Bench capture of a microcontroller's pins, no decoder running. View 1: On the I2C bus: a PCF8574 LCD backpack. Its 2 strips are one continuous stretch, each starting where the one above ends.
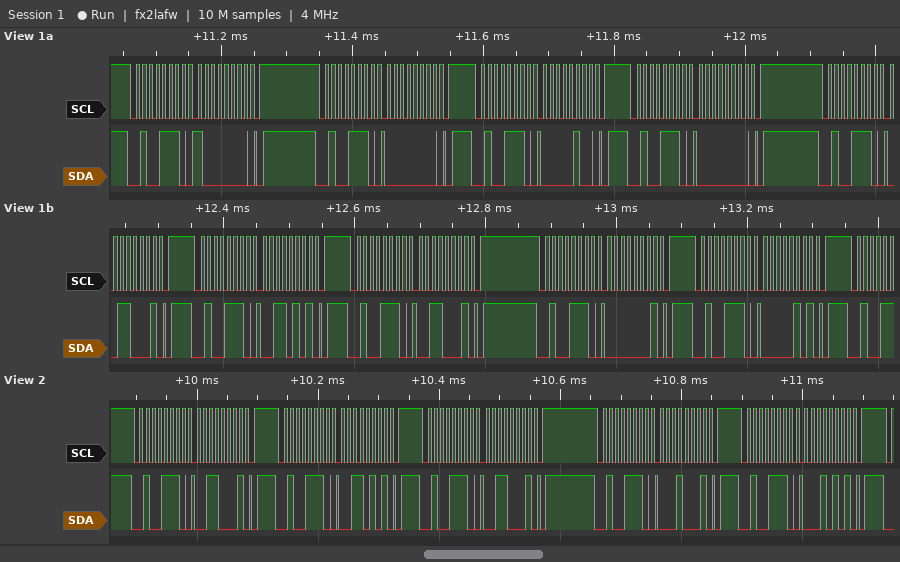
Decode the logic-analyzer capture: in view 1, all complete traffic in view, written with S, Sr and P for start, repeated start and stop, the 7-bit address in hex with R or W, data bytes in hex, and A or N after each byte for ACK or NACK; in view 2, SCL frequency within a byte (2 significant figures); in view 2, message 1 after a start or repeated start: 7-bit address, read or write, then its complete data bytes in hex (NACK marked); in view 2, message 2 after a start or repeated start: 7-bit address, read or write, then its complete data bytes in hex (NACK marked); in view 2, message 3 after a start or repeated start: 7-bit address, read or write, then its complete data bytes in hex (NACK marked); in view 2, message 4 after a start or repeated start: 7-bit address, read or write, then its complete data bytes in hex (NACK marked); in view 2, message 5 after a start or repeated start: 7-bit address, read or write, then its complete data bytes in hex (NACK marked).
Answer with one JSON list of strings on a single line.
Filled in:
["S 27W A 80 A P S 27W A 00 A P S 27W A 04 A P S 27W A 00 A P S 27W A 31 A P S 27W A 35 A P S 27W A 31 A P S 27W A 01 A P S 27W A 05 A P", "100 kHz", "0x27 write: 31", "0x27 write: 35", "0x27 write: 31", "0x27 write: 11", "0x27 write: 15"]
